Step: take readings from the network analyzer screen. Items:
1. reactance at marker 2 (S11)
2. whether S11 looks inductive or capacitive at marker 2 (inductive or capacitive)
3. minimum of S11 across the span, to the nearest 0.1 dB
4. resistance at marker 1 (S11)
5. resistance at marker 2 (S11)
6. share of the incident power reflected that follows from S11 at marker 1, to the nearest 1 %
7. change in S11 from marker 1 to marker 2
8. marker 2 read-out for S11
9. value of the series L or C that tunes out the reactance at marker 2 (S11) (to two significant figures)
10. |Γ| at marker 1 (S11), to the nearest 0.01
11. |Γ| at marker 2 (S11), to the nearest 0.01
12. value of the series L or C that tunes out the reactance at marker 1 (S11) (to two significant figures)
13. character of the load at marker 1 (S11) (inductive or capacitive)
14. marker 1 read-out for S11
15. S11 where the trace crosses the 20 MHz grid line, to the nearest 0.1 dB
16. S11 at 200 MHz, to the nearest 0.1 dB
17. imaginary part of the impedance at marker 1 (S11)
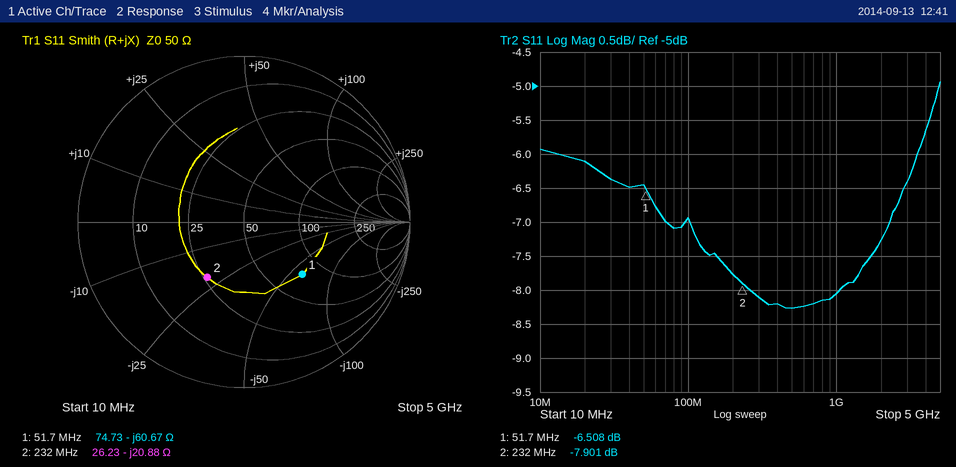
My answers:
-20.88 Ω
capacitive
-8.3 dB
74.73 Ω
26.23 Ω
22 %
-1.393 dB
-7.901 dB
14 nH
0.47
0.40
190 nH
capacitive
-6.508 dB
-6.1 dB
-7.8 dB
-60.67 Ω
